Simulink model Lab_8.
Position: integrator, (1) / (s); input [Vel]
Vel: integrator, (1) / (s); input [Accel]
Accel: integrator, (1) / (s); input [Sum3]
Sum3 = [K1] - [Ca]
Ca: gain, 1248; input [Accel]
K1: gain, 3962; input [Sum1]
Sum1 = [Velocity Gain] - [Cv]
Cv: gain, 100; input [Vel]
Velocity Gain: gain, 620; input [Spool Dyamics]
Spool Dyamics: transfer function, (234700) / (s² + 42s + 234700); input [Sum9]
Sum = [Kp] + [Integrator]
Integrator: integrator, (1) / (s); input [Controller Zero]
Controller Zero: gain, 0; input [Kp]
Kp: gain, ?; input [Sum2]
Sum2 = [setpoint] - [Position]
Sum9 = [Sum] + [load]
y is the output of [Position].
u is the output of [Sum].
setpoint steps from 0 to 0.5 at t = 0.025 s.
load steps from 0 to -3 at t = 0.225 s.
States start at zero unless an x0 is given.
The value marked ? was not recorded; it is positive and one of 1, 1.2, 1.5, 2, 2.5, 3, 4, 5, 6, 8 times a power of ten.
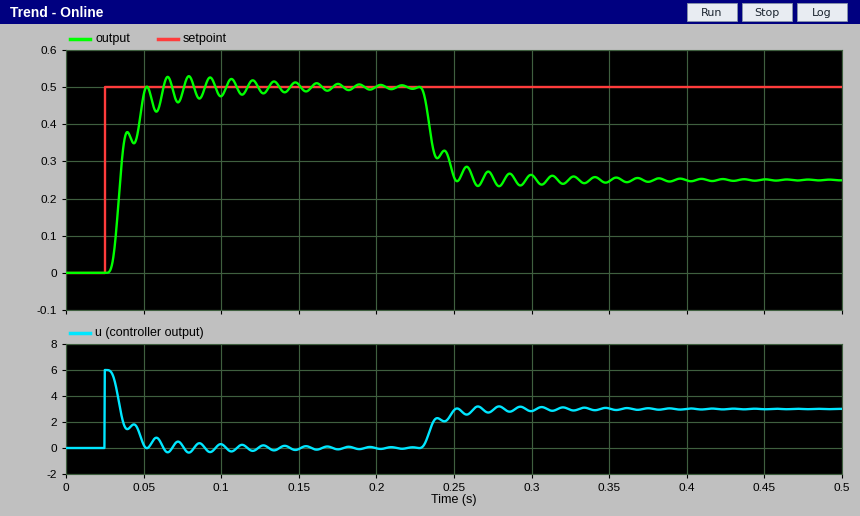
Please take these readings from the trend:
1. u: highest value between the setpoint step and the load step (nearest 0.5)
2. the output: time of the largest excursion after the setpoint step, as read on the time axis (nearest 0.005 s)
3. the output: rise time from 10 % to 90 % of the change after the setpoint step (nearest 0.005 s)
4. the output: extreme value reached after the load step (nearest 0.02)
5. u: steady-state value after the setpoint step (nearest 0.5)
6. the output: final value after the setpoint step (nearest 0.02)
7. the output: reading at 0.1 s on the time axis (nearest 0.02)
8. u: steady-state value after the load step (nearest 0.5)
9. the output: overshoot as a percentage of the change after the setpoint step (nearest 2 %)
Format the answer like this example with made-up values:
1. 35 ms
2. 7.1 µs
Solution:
1. 6.0
2. 0.080 s
3. 0.020 s
4. 0.24
5. 0.0
6. 0.50
7. 0.48
8. 3.0
9. 6 %
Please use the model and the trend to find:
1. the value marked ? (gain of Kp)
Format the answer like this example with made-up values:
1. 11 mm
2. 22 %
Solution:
1. 12
